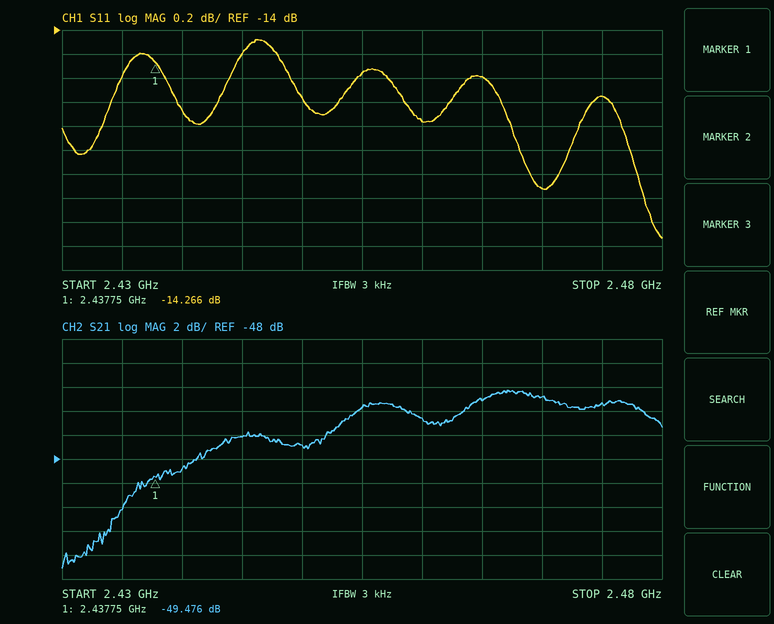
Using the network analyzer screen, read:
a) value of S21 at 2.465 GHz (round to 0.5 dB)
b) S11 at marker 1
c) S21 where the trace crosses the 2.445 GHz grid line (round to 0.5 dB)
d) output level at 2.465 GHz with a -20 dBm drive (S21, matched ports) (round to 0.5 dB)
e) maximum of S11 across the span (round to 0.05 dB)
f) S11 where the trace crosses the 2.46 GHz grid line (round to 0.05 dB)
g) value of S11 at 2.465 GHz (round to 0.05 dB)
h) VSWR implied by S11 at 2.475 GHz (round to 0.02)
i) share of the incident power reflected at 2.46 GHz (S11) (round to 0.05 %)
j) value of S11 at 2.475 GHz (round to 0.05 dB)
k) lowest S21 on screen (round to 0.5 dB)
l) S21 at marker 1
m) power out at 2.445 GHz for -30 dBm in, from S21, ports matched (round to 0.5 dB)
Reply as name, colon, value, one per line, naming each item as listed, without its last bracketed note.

value of S21 at 2.465 GHz: -43.0 dB
S11 at marker 1: -14.266 dB
S21 where the trace crosses the 2.445 GHz grid line: -46.0 dB
output level at 2.465 GHz with a -20 dBm drive (S21, matched ports): -63.0 dBm
maximum of S11 across the span: -14.10 dB
S11 where the trace crosses the 2.46 GHz grid line: -14.75 dB
value of S11 at 2.465 GHz: -14.40 dB
VSWR implied by S11 at 2.475 GHz: 1.46
share of the incident power reflected at 2.46 GHz (S11): 3.35 %
value of S11 at 2.475 GHz: -14.55 dB
lowest S21 on screen: -57.0 dB
S21 at marker 1: -49.476 dB
power out at 2.445 GHz for -30 dBm in, from S21, ports matched: -76.0 dBm
